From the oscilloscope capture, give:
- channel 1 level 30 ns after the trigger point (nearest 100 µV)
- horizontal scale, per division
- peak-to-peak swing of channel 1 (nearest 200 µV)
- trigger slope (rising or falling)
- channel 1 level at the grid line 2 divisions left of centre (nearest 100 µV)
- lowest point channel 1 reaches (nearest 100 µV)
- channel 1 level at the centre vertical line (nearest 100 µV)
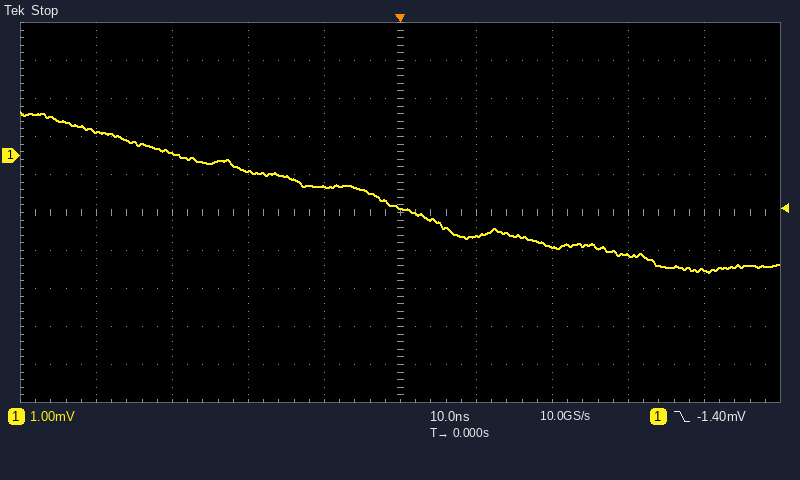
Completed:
-2.6 mV
10 ns
4.2 mV
falling
-400 µV
-3.1 mV
-1.4 mV
